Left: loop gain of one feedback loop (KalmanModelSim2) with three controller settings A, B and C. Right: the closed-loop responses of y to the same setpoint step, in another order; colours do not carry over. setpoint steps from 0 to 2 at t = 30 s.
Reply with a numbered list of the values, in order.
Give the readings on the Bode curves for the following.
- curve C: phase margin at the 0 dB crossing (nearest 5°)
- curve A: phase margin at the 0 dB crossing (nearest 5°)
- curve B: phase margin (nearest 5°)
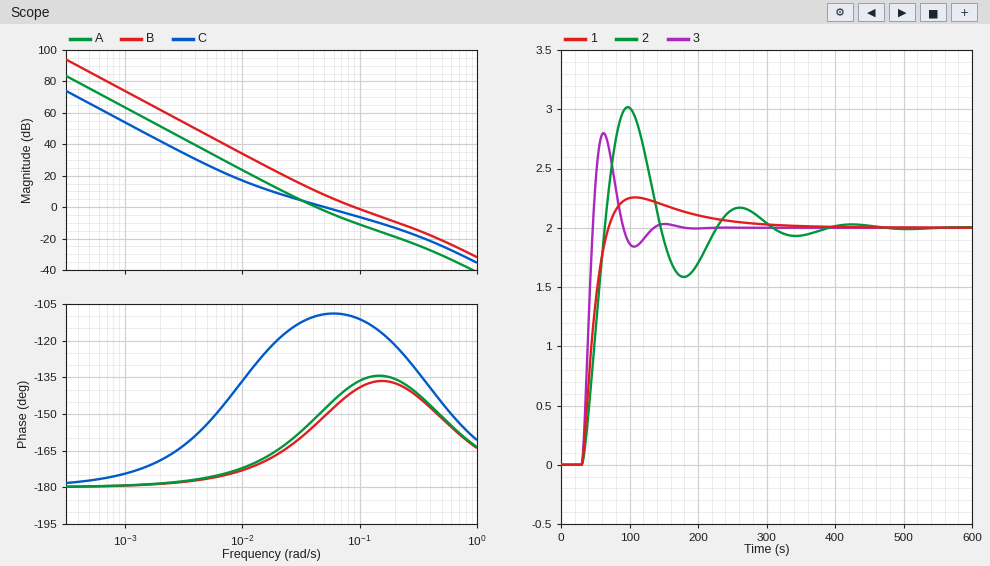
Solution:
1. 70°
2. 30°
3. 40°
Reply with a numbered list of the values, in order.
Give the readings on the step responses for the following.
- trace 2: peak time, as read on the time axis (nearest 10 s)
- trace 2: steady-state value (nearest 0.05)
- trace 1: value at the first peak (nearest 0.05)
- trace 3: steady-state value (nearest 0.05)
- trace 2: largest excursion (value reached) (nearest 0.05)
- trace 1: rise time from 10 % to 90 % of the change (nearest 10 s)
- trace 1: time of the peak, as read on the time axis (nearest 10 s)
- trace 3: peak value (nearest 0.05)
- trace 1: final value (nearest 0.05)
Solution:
1. 100 s
2. 2.00
3. 2.25
4. 2.00
5. 3.00
6. 30 s
7. 110 s
8. 2.80
9. 2.00
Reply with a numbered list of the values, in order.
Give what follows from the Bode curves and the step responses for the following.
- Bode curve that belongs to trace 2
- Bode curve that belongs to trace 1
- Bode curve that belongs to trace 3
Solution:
1. A
2. C
3. B
